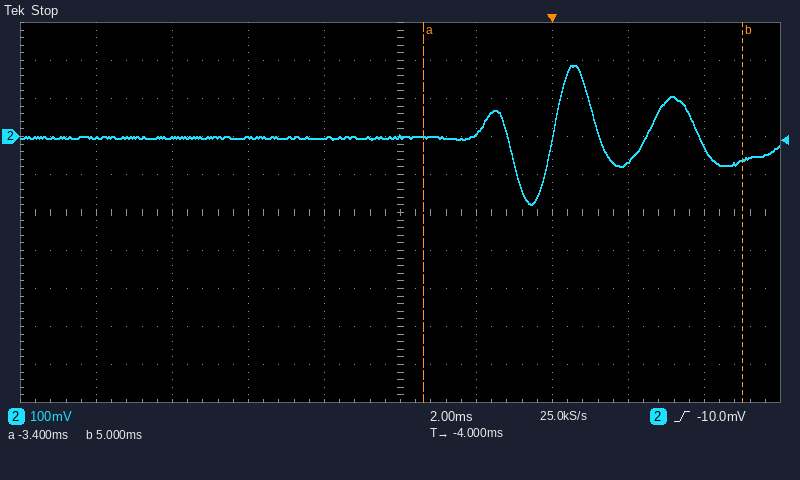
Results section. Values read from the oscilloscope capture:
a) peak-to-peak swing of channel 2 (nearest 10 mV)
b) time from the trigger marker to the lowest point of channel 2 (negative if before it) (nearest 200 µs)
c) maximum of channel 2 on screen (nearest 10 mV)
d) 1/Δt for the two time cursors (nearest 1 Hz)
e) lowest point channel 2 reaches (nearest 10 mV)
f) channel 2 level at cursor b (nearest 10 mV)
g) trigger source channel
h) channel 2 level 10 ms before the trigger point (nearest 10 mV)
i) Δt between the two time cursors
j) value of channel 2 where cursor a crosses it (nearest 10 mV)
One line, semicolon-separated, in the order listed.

370 mV; -600 µs; 190 mV; 119 Hz; -180 mV; -60 mV; channel 2; 0 mV; 8.4 ms; 0 mV
